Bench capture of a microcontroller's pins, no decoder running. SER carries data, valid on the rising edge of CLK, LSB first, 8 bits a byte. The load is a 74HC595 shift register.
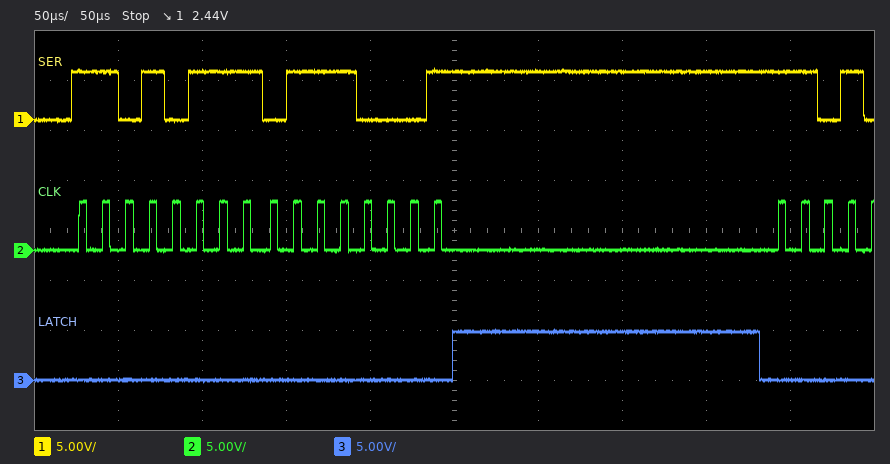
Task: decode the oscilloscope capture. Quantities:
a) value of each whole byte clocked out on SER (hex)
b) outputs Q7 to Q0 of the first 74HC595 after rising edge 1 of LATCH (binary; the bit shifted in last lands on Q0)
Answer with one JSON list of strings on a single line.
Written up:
["EB 8E", "01110001"]
